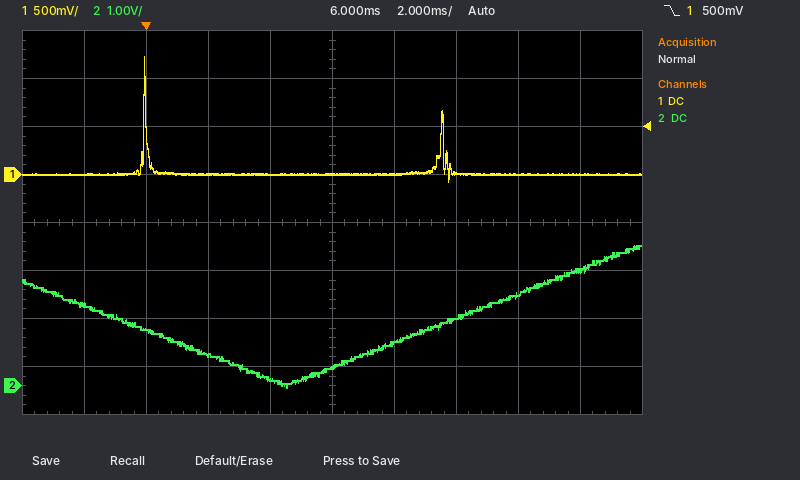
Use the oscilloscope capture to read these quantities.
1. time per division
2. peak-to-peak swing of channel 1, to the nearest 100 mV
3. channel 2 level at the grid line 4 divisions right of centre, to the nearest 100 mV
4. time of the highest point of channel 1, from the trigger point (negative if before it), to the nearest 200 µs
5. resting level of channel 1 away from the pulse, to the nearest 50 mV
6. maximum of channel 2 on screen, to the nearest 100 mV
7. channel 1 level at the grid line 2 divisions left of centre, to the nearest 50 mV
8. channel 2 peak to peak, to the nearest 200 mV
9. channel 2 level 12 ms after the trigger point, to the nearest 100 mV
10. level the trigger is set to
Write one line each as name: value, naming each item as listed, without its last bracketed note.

time per division: 2 ms
peak-to-peak swing of channel 1, to the nearest 100 mV: 1.30 V
channel 2 level at the grid line 4 divisions right of centre, to the nearest 100 mV: 2.4 V
time of the highest point of channel 1, from the trigger point (negative if before it), to the nearest 200 µs: 0.0 ms
resting level of channel 1 away from the pulse, to the nearest 50 mV: 0 mV
maximum of channel 2 on screen, to the nearest 100 mV: 2.9 V
channel 1 level at the grid line 2 divisions left of centre, to the nearest 50 mV: 0 mV
channel 2 peak to peak, to the nearest 200 mV: 3.0 V
channel 2 level 12 ms after the trigger point, to the nearest 100 mV: 1.9 V
level the trigger is set to: 500 mV
